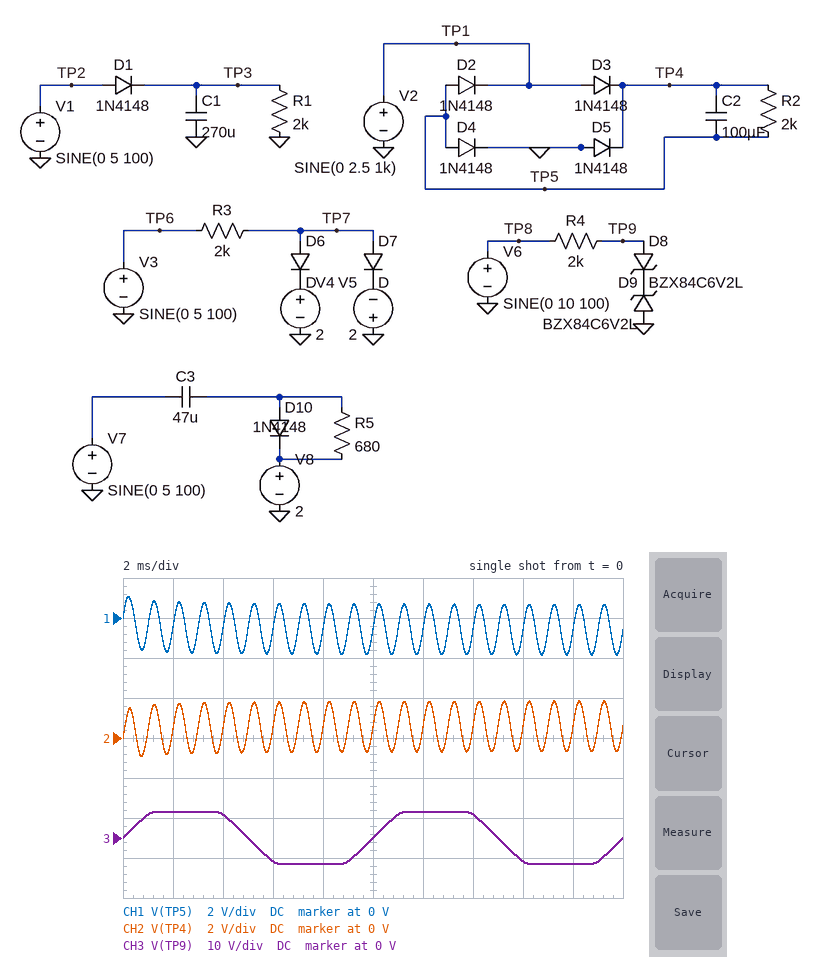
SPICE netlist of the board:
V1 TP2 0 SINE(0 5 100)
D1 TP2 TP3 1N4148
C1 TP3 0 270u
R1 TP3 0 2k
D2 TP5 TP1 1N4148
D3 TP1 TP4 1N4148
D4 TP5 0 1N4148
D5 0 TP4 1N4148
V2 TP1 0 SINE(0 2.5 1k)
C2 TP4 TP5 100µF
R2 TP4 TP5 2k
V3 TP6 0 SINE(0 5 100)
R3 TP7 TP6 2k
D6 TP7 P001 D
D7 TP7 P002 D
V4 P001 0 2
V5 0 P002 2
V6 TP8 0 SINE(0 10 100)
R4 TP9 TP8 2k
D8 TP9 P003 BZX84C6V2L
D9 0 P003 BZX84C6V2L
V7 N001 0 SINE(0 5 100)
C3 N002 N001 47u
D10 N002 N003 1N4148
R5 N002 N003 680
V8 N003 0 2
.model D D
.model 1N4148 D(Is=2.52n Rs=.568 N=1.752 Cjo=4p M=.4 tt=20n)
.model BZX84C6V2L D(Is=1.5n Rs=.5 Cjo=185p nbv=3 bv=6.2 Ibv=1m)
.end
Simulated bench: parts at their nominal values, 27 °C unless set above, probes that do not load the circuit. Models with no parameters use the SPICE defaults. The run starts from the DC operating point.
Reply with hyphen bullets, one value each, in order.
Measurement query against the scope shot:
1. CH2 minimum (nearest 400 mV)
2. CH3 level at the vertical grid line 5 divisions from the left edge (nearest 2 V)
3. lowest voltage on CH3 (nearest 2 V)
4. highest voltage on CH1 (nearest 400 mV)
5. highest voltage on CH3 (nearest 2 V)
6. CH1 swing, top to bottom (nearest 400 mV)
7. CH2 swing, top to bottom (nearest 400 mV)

- -800 mV
- 0 V
- -6 V
- 1.2 V
- 6 V
- 2.8 V
- 2.8 V
